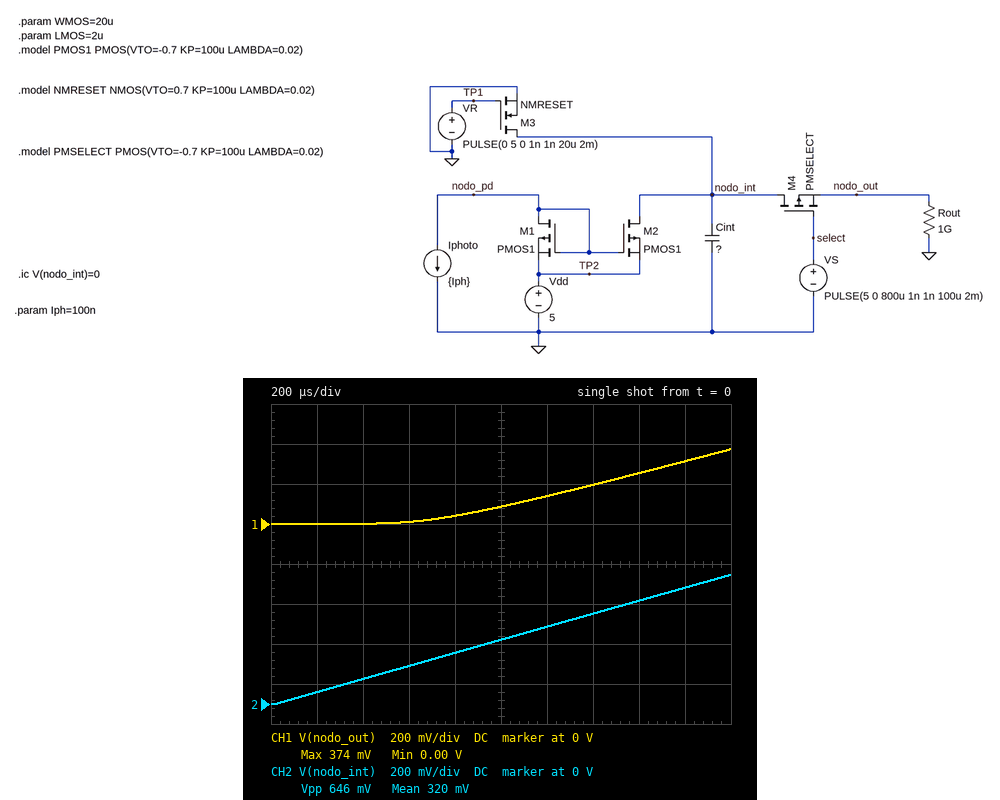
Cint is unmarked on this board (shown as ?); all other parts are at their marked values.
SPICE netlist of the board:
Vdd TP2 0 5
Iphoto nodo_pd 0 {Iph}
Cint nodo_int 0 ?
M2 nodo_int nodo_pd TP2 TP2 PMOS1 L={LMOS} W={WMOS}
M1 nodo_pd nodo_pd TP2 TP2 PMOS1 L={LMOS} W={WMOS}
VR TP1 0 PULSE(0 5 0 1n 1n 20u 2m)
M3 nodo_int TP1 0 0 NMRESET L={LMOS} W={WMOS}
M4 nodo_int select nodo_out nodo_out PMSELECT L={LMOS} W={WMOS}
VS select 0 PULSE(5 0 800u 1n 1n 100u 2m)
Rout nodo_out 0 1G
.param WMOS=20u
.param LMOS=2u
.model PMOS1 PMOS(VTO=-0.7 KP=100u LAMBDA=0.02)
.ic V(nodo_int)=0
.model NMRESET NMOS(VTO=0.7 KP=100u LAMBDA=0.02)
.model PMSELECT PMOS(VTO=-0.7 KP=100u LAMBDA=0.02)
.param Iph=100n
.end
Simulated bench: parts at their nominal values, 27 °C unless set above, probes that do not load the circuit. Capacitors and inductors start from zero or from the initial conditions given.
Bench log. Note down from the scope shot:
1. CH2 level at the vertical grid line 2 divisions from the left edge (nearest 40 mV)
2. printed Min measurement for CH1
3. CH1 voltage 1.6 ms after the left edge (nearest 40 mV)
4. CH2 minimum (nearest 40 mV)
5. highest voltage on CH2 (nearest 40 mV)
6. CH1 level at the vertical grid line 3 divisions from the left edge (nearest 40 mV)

120 mV
0.00 V
240 mV
0 V
640 mV
0 V
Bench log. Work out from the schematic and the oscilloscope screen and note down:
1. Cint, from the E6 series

330 pF
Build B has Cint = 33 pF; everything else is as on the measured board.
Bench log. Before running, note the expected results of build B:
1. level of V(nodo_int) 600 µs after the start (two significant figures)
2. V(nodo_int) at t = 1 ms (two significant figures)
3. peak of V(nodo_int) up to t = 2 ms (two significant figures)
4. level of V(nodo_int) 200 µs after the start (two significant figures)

1.9 V
3.1 V
5.0 V
590 mV
